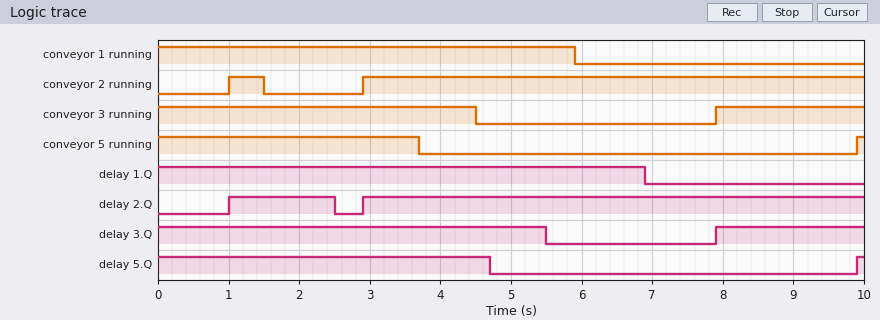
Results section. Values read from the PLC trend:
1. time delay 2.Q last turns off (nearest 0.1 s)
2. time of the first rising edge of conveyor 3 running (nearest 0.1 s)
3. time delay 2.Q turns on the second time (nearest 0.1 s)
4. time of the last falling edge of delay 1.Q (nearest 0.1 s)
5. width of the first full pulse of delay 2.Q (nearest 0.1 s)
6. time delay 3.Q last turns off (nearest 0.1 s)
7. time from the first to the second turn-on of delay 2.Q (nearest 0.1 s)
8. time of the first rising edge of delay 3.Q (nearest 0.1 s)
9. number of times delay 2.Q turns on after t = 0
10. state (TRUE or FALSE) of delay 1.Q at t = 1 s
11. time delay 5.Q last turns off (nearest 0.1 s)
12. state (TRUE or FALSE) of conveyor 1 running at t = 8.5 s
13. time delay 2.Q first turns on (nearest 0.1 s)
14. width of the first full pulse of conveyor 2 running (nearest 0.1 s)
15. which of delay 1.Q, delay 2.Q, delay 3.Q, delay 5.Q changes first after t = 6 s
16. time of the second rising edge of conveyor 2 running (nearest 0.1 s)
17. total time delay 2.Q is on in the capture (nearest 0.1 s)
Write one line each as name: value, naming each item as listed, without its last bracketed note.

time delay 2.Q last turns off: 2.5 s
time of the first rising edge of conveyor 3 running: 7.9 s
time delay 2.Q turns on the second time: 2.9 s
time of the last falling edge of delay 1.Q: 6.9 s
width of the first full pulse of delay 2.Q: 1.5 s
time delay 3.Q last turns off: 5.5 s
time from the first to the second turn-on of delay 2.Q: 1.9 s
time of the first rising edge of delay 3.Q: 7.9 s
number of times delay 2.Q turns on after t = 0: 2
state (TRUE or FALSE) of delay 1.Q at t = 1 s: TRUE
time delay 5.Q last turns off: 4.7 s
state (TRUE or FALSE) of conveyor 1 running at t = 8.5 s: FALSE
time delay 2.Q first turns on: 1.0 s
width of the first full pulse of conveyor 2 running: 0.5 s
which of delay 1.Q, delay 2.Q, delay 3.Q, delay 5.Q changes first after t = 6 s: delay 1.Q
time of the second rising edge of conveyor 2 running: 2.9 s
total time delay 2.Q is on in the capture: 8.6 s
